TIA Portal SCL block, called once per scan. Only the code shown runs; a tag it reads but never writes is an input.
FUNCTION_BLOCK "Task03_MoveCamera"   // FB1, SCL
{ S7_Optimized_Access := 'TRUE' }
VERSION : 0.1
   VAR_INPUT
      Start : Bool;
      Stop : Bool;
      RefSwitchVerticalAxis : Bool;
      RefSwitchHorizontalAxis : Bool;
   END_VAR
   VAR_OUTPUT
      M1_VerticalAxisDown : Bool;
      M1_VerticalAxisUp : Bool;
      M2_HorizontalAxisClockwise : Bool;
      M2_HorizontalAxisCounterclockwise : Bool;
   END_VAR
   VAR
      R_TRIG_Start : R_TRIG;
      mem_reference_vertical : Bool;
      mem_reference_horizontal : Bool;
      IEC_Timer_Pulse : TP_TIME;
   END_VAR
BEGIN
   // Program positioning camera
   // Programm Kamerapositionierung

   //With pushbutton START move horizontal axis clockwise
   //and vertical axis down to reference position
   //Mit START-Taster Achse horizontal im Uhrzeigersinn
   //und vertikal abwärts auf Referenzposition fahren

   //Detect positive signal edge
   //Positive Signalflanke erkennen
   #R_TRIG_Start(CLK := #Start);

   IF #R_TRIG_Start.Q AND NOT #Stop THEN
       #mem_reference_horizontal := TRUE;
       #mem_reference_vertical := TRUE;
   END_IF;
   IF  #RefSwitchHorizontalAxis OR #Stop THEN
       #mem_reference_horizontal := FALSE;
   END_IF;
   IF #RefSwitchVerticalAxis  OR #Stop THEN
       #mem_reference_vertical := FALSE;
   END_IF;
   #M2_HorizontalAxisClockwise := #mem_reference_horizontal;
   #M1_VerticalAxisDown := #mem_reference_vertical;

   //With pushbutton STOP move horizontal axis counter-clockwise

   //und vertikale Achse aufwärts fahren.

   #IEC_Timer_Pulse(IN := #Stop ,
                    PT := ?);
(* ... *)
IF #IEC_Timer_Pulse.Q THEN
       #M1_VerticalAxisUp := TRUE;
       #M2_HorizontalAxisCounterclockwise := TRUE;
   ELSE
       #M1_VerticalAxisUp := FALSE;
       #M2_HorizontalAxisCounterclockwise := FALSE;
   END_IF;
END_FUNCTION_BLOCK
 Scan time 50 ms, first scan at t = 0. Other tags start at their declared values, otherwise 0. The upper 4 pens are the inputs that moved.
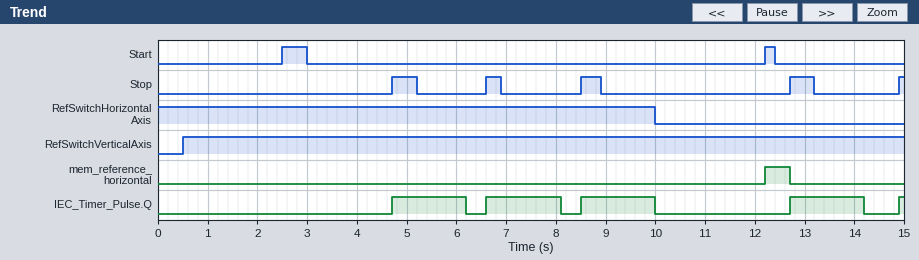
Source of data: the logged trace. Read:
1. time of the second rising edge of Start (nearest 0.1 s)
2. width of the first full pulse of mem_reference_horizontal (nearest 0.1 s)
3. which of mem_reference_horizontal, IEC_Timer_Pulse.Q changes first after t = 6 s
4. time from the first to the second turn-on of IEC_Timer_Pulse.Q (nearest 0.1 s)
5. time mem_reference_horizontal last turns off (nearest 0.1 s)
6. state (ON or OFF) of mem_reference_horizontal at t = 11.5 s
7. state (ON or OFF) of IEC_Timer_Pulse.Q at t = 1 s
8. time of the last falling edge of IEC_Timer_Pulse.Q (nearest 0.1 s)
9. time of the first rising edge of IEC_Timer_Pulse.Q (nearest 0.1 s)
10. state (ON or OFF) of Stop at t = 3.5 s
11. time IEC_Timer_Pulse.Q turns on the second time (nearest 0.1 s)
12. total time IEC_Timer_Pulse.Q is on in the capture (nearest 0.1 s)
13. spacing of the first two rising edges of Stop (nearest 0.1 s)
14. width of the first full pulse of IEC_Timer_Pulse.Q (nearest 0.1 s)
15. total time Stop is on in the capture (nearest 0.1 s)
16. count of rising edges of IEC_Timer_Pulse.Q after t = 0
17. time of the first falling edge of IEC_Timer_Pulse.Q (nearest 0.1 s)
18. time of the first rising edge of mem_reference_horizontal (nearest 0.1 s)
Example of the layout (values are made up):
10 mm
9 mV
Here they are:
12.2 s
0.5 s
IEC_Timer_Pulse.Q
1.9 s
12.7 s
OFF
OFF
14.2 s
4.7 s
OFF
6.6 s
6.1 s
1.9 s
1.5 s
1.8 s
5
6.2 s
12.2 s
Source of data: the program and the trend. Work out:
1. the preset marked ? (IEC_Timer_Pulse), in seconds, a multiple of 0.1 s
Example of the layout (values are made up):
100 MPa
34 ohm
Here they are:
1.5 s
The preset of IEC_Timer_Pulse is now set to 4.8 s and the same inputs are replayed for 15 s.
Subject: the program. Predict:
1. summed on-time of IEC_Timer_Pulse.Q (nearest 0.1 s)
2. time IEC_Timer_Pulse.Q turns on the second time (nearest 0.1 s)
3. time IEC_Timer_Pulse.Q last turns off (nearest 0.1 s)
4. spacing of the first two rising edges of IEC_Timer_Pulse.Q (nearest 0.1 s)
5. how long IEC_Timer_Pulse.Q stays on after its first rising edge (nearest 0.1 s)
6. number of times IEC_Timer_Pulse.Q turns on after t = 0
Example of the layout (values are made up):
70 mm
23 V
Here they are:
7.1 s
12.7 s
9.5 s
8.0 s
4.8 s
2
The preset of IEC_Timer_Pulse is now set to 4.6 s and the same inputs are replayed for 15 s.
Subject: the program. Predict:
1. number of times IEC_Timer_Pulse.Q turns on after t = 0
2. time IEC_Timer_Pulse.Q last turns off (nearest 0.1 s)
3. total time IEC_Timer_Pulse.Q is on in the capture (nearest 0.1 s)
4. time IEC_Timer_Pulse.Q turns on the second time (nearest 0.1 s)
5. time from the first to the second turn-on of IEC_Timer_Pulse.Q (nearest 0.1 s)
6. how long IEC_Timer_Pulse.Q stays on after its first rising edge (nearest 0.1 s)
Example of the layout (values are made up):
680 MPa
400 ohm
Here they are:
2
9.3 s
6.9 s
12.7 s
8.0 s
4.6 s
